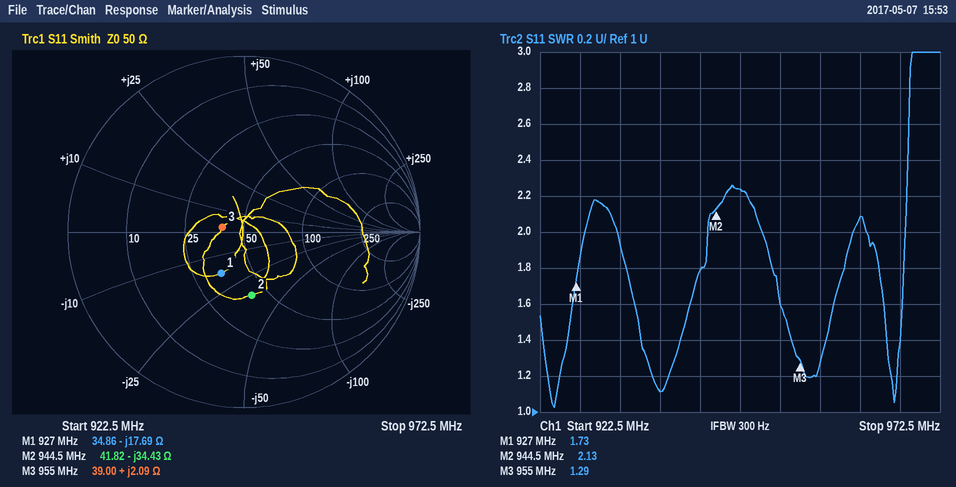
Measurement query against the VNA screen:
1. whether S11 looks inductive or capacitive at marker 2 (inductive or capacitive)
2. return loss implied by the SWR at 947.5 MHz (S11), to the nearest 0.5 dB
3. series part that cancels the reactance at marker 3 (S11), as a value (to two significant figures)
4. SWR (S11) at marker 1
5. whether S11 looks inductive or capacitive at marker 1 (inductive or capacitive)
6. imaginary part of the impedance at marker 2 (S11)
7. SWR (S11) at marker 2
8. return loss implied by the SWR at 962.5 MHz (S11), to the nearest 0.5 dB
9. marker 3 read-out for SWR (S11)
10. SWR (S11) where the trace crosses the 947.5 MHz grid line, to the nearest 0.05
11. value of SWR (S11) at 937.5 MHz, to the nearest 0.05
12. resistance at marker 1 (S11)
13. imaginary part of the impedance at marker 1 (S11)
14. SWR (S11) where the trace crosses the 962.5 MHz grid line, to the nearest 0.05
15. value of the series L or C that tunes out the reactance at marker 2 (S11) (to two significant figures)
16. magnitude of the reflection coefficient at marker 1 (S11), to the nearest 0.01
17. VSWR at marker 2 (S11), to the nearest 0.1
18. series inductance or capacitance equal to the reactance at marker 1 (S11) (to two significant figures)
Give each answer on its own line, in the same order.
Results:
capacitive
8.5 dB
80 pF
1.73
capacitive
-34.43 Ω
2.13
9.0 dB
1.29
2.25
1.10
34.86 Ω
-17.69 Ω
2.10
5.8 nH
0.27
2.1
9.7 pF
